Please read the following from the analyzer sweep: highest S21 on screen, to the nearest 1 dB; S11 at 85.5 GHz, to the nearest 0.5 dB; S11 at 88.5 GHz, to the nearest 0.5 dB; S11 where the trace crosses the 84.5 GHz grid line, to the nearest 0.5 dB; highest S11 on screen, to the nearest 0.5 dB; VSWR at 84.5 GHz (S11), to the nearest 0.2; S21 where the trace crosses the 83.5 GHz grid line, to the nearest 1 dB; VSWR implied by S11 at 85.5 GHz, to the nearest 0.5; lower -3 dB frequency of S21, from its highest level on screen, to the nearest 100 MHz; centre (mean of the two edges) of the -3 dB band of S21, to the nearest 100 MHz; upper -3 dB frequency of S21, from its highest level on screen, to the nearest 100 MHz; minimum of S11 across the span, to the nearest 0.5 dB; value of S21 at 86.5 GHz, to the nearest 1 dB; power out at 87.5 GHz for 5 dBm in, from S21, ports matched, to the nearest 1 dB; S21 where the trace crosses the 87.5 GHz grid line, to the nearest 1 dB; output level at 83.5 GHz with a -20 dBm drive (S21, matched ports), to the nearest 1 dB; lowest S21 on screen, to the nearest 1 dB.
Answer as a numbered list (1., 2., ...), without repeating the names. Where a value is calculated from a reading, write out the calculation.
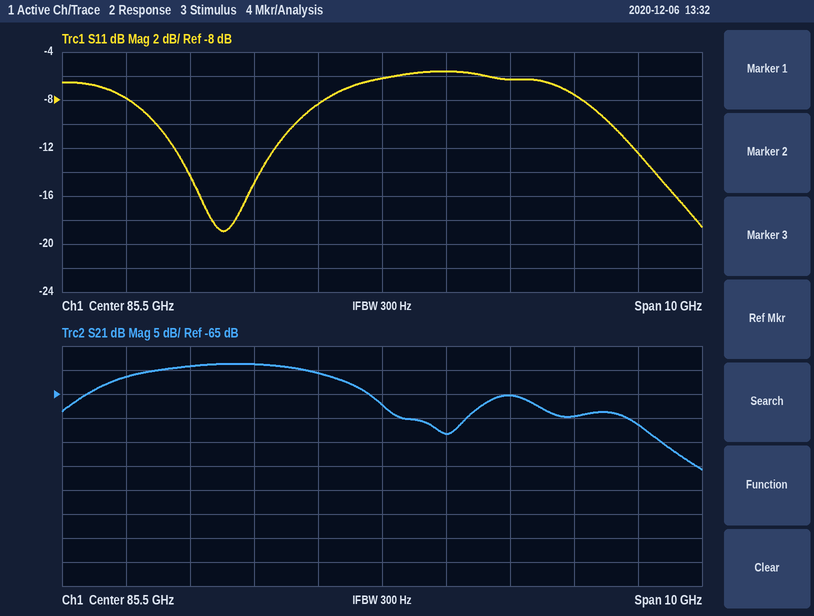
1. -59 dB
2. -6.0 dB
3. -7.5 dB
4. -8.5 dB
5. -5.5 dB
6. |Γ| = 10^(-8.5/20) = 0.3758; VSWR = (1 + 0.3758)/(1 − 0.3758) ≈ 2.2
7. -59 dB
8. |Γ| = 10^(-6/20) = 0.5012; VSWR = (1 + 0.5012)/(1 − 0.5012) ≈ 3.0
9. 81.4 GHz
10. 83.1 GHz
11. 84.8 GHz
12. -19.0 dB
13. -73 dB
14. 5 dBm + (-65 dB) = -60 dBm
15. -65 dB
16. -20 dBm + (-59 dB) = -79 dBm
17. -81 dB
